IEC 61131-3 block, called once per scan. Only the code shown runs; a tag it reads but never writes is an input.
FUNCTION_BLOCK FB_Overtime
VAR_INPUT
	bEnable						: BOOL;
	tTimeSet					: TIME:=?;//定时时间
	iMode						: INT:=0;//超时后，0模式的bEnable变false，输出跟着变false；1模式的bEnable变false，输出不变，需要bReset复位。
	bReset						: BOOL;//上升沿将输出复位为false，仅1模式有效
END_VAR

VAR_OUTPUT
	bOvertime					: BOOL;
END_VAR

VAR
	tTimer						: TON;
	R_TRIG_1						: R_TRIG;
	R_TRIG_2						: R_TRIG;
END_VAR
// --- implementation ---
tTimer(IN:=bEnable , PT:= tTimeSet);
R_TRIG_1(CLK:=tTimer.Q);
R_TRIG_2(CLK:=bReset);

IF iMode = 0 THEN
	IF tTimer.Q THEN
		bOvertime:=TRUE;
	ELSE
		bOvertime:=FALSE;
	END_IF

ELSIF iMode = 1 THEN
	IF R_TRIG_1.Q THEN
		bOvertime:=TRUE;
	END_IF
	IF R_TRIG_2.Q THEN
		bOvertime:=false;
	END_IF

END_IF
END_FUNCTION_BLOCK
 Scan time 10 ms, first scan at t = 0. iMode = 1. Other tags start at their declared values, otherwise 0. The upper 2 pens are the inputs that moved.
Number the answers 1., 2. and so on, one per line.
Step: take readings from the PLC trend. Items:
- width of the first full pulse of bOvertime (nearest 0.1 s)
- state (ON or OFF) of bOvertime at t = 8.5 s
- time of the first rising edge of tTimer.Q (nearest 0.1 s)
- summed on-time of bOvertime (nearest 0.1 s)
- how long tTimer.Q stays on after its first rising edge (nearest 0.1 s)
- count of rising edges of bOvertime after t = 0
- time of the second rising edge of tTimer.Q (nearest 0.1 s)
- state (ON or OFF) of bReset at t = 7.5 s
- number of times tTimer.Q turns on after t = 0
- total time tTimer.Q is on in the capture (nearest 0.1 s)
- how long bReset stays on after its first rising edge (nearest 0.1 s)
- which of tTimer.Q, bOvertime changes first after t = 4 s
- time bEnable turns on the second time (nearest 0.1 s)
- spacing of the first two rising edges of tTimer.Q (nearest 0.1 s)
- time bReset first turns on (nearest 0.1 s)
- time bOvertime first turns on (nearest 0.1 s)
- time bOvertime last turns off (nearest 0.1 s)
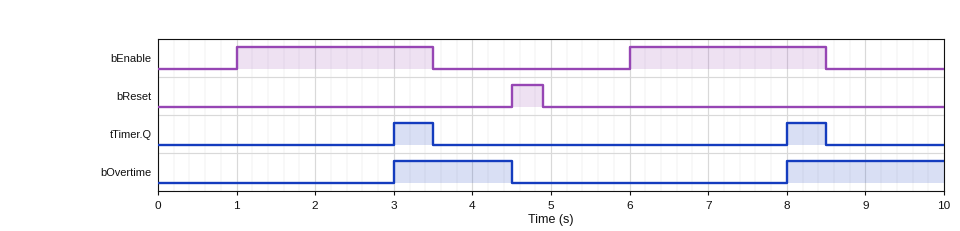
1. 1.5 s
2. ON
3. 3.0 s
4. 3.5 s
5. 0.5 s
6. 2
7. 8.0 s
8. OFF
9. 2
10. 1.0 s
11. 0.4 s
12. bOvertime
13. 6.0 s
14. 5.0 s
15. 4.5 s
16. 3.0 s
17. 4.5 s
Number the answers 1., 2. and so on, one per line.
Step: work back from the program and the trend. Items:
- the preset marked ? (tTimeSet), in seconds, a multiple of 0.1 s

1. 2.0 s
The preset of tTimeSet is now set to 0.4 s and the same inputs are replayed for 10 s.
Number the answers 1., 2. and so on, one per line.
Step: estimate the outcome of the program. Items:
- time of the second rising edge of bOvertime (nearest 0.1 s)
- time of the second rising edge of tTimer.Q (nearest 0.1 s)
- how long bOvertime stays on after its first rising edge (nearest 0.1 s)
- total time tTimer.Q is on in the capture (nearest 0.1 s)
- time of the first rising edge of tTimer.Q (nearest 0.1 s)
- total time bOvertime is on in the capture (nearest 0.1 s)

1. 6.4 s
2. 6.4 s
3. 3.1 s
4. 4.2 s
5. 1.4 s
6. 6.7 s
